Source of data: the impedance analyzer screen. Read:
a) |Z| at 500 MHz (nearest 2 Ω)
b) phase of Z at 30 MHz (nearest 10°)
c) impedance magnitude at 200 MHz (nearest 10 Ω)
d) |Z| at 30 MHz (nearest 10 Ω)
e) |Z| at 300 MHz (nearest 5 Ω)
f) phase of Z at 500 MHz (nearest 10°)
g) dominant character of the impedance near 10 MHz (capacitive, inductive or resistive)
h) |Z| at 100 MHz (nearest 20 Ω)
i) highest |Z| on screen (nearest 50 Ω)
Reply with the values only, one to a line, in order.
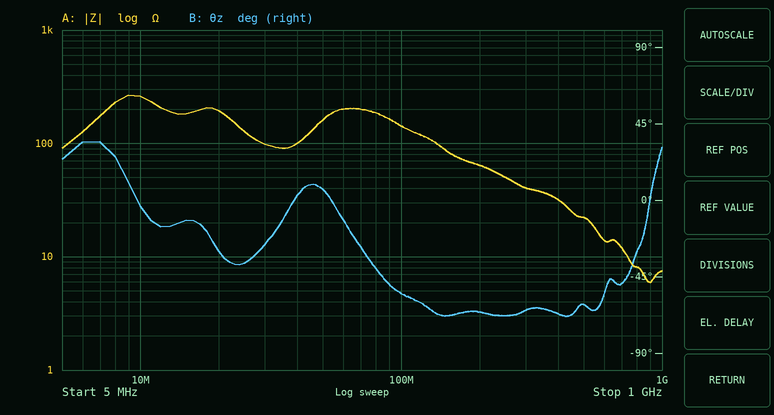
22 Ω
-30°
60 Ω
100 Ω
40 Ω
-60°
resistive
140 Ω
250 Ω
